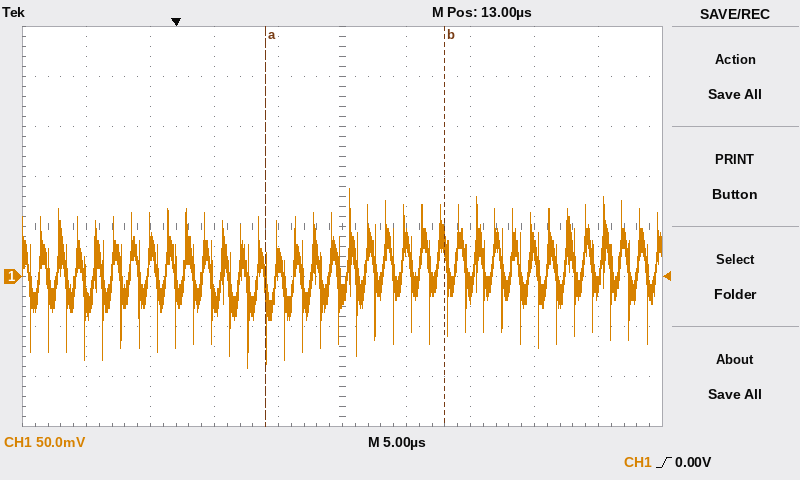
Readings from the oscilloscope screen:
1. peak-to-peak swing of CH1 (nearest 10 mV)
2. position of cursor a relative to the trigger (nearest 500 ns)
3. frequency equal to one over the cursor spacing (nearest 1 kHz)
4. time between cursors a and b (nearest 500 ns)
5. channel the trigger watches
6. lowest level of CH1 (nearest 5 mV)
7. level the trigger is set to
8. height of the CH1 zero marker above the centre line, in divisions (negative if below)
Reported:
180 mV
+7.0 µs
71 kHz
14.0 µs
CH1
-90 mV
0.00 V
-1.0 div
